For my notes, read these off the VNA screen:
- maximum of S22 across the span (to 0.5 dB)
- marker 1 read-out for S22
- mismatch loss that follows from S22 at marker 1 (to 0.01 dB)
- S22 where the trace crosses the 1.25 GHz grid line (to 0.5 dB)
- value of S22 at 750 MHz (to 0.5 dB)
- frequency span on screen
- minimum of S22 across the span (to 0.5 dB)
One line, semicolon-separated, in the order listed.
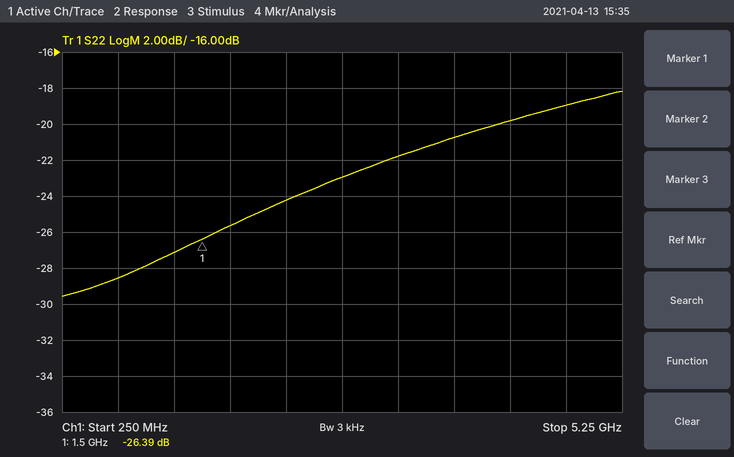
-18.0 dB; -26.39 dB; 0.01 dB; -27.0 dB; -28.5 dB; 5 GHz; -29.5 dB
